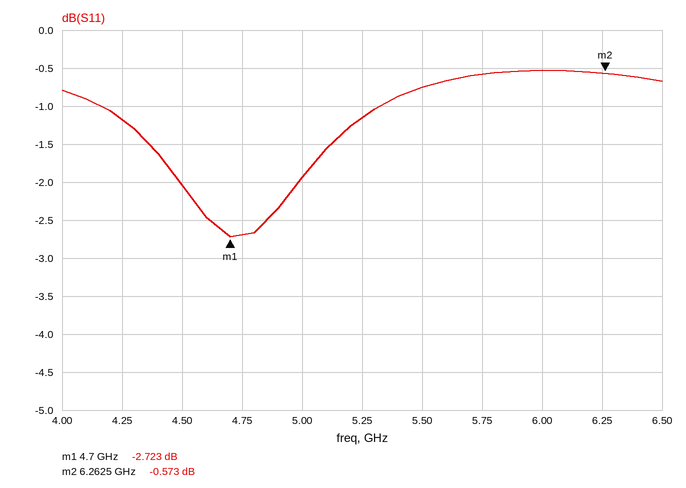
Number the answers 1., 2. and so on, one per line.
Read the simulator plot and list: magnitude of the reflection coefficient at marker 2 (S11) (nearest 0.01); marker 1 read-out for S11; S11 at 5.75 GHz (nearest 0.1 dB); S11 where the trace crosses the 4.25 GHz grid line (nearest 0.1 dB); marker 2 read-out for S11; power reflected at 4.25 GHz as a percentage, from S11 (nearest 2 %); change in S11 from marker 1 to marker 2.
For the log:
1. 0.94
2. -2.723 dB
3. -0.6 dB
4. -1.2 dB
5. -0.573 dB
6. 76 %
7. 2.150 dB
